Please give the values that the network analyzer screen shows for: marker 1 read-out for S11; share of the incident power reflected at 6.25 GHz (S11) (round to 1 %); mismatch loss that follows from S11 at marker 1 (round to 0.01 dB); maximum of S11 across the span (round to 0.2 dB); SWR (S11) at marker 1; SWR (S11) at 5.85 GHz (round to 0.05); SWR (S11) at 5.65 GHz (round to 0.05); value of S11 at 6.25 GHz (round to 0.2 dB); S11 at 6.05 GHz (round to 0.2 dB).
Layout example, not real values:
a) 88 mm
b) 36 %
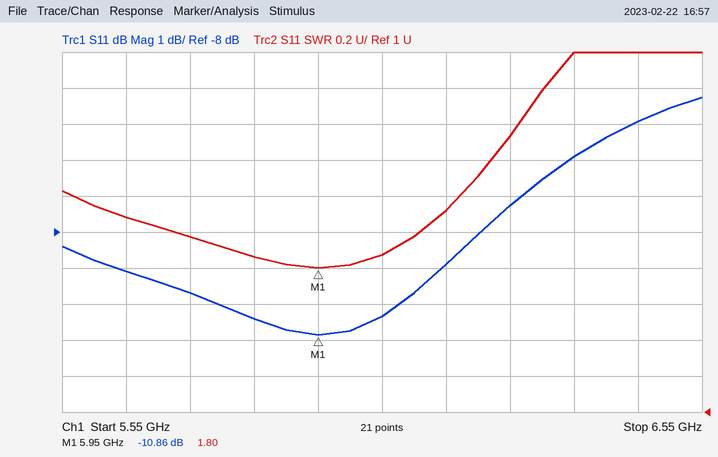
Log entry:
a) -10.86 dB
b) 19 %
c) 0.37 dB
d) -4.2 dB
e) 1.80
f) 1.85
g) 2.10
h) -7.2 dB
i) -10.4 dB
